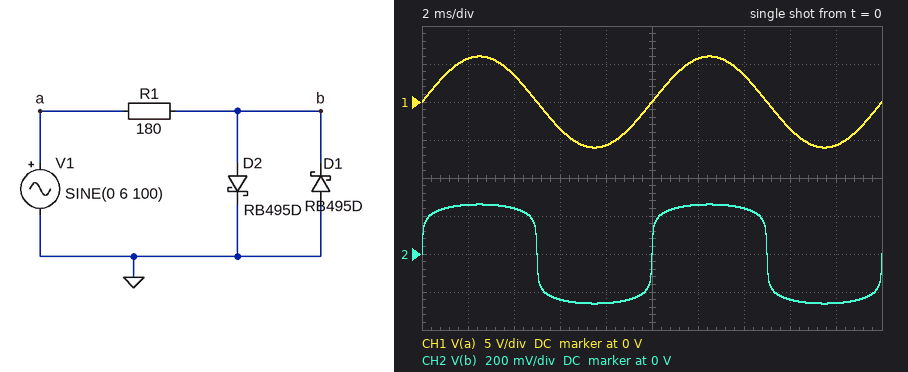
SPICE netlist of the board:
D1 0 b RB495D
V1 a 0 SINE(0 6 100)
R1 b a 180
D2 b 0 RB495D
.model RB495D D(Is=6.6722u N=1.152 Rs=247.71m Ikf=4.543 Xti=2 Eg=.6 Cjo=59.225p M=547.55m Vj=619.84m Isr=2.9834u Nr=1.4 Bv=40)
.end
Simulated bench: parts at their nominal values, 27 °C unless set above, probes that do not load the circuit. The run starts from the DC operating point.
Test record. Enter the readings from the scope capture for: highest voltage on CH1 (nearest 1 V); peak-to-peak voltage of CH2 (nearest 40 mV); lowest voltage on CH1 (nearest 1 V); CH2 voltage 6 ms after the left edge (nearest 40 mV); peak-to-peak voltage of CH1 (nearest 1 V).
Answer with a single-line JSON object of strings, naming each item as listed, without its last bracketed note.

{"highest voltage on CH1": "6 V", "peak-to-peak voltage of CH2": "520 mV", "lowest voltage on CH1": "-6 V", "CH2 voltage 6 ms after the left edge": "-240 mV", "peak-to-peak voltage of CH1": "12 V"}
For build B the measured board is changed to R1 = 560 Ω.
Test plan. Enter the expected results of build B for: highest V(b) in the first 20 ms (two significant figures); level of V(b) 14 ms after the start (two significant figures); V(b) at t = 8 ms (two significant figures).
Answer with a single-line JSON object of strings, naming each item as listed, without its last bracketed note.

{"highest V(b) in the first 20 ms": "220 mV", "level of V(b) 14 ms after the start": "200 mV", "V(b) at t = 8 ms": "-220 mV"}
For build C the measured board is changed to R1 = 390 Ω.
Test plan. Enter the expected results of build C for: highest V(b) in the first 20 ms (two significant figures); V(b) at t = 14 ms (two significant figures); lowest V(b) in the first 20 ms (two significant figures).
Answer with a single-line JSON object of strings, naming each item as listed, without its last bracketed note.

{"highest V(b) in the first 20 ms": "230 mV", "V(b) at t = 14 ms": "210 mV", "lowest V(b) in the first 20 ms": "-230 mV"}
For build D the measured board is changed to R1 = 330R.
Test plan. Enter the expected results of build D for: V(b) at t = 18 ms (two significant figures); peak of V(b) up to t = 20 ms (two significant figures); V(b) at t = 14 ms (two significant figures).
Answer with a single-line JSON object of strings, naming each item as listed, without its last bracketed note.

{"V(b) at t = 18 ms": "-240 mV", "peak of V(b) up to t = 20 ms": "240 mV", "V(b) at t = 14 ms": "220 mV"}
